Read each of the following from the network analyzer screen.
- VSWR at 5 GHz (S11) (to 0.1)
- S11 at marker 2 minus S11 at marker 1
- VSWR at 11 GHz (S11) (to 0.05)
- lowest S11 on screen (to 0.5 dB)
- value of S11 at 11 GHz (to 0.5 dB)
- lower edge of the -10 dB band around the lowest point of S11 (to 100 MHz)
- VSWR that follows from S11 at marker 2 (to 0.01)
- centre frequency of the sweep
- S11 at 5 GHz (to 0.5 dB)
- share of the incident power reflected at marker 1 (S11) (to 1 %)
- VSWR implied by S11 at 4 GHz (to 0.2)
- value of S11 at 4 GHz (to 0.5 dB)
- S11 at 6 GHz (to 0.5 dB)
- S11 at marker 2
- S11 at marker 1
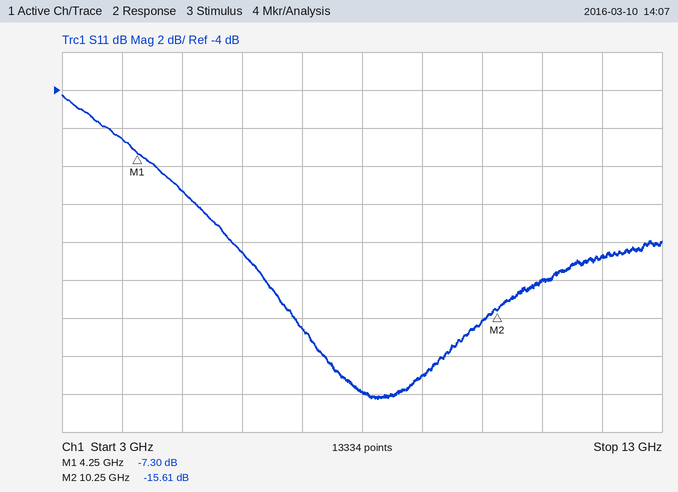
2.0
-8.31 dB
1.50
-20.5 dB
-14.0 dB
5.2 GHz
1.40
8 GHz
-9.5 dB
19 %
2.8
-6.5 dB
-12.5 dB
-15.61 dB
-7.30 dB
